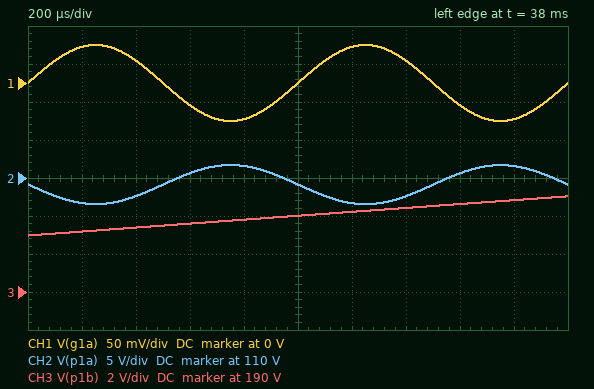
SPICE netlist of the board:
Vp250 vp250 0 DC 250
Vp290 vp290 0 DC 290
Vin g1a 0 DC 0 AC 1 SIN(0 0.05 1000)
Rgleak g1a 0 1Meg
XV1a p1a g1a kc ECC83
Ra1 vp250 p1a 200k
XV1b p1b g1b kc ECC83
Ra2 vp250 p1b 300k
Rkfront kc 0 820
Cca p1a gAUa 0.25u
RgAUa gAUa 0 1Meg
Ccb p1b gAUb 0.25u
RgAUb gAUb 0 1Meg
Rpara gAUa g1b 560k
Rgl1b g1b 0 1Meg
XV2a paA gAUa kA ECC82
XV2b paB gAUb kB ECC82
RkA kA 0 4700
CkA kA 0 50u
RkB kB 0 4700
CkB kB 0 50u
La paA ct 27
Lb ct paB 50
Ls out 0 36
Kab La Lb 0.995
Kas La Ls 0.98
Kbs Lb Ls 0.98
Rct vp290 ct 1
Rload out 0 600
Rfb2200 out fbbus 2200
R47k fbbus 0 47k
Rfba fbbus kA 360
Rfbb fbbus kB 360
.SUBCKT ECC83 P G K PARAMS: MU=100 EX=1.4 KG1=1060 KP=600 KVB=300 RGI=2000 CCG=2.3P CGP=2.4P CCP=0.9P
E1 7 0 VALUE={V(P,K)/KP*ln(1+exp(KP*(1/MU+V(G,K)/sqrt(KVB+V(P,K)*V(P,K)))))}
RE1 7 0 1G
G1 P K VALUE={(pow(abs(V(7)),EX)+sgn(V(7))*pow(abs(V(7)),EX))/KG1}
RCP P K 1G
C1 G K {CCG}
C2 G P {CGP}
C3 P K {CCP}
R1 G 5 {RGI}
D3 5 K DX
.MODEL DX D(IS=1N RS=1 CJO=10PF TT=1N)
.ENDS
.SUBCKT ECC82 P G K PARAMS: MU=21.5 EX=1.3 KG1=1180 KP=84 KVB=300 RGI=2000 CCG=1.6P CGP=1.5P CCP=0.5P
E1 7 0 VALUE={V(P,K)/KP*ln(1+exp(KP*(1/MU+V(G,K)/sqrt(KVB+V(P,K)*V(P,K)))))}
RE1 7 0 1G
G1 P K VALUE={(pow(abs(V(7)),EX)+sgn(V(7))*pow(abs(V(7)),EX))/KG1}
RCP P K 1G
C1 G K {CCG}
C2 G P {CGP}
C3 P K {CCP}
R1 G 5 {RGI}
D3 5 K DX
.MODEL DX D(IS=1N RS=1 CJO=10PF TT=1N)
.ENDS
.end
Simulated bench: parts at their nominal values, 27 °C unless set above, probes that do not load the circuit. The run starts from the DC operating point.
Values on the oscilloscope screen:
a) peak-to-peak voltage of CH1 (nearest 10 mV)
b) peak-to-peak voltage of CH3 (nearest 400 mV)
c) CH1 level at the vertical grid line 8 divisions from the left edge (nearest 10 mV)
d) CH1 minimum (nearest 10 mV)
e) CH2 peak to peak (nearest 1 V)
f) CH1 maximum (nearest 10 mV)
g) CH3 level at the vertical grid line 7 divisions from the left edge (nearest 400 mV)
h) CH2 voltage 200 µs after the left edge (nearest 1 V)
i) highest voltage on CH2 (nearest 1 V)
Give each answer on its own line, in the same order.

100 mV
2.0 V
-30 mV
-50 mV
5 V
50 mV
194.4 V
107 V
112 V
